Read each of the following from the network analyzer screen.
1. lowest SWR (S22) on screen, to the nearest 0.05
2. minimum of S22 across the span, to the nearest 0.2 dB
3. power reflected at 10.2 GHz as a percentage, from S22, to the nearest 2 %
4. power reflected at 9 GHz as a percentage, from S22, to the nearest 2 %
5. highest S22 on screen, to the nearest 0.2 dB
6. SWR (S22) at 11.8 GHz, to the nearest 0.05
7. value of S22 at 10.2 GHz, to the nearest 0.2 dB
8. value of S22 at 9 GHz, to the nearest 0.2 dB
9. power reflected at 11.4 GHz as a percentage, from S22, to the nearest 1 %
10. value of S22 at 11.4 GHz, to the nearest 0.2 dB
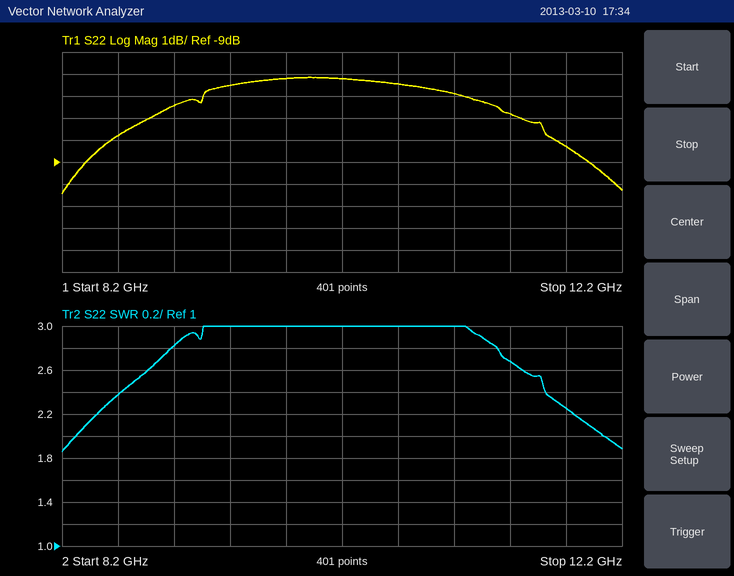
1.85
-10.4 dB
30 %
22 %
-5.2 dB
2.25
-5.2 dB
-6.4 dB
21 %
-6.8 dB
